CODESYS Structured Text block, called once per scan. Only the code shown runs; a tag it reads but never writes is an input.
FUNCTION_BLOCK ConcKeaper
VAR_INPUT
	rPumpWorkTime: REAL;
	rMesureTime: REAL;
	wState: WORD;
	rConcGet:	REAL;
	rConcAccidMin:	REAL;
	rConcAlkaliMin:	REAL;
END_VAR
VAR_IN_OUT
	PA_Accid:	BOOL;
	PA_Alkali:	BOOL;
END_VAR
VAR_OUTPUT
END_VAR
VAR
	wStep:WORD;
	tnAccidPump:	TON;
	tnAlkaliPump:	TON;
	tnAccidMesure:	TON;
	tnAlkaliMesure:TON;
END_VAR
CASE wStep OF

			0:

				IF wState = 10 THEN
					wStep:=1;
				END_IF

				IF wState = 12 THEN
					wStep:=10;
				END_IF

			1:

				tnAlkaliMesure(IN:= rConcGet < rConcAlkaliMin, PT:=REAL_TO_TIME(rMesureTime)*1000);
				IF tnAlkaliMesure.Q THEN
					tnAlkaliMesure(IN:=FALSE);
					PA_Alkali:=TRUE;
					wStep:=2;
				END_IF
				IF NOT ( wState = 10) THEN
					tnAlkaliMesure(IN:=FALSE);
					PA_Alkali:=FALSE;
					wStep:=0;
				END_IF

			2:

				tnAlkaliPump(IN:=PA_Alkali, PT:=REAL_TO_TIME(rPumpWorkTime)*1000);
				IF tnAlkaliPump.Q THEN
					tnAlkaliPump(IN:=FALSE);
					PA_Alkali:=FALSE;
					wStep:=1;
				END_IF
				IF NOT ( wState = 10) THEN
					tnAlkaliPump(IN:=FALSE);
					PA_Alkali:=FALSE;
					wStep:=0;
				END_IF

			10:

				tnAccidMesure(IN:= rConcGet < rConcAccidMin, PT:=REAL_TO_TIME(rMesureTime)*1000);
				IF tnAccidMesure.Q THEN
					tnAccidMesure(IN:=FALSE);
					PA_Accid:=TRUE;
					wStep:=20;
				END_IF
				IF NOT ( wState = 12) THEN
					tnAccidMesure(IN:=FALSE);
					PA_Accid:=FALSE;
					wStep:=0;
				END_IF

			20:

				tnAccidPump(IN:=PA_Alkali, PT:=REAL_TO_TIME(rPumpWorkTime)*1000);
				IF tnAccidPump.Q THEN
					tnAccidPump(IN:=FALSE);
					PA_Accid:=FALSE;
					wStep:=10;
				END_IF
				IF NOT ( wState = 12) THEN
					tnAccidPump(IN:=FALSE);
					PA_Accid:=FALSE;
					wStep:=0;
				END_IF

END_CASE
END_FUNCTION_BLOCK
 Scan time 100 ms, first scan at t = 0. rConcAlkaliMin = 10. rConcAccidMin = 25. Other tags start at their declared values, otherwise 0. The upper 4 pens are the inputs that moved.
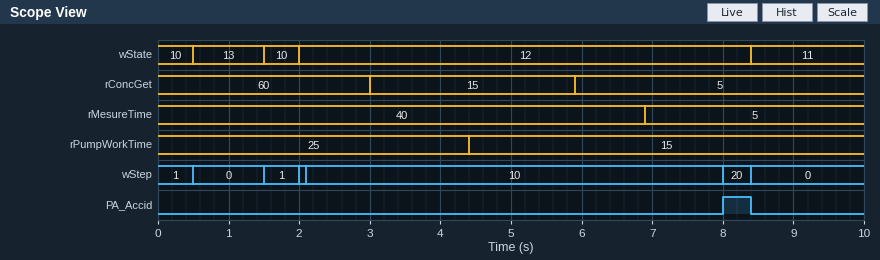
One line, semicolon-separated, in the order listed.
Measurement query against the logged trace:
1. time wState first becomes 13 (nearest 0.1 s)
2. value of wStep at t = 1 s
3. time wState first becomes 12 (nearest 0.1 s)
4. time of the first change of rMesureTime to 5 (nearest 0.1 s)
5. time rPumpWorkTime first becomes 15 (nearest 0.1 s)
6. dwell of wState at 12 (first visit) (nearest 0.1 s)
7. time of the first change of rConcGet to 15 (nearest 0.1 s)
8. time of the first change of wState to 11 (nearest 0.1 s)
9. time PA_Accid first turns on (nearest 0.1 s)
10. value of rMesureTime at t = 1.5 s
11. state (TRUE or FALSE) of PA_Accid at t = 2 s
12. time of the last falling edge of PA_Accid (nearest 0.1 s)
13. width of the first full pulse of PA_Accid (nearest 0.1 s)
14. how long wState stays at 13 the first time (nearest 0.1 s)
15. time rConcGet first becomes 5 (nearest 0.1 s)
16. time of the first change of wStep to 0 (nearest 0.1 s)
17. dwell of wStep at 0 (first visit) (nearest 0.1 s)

0.5 s; 0; 2.0 s; 6.9 s; 4.4 s; 6.4 s; 3.0 s; 8.4 s; 8.0 s; 40; FALSE; 8.4 s; 0.4 s; 1.0 s; 5.9 s; 0.5 s; 1.0 s
